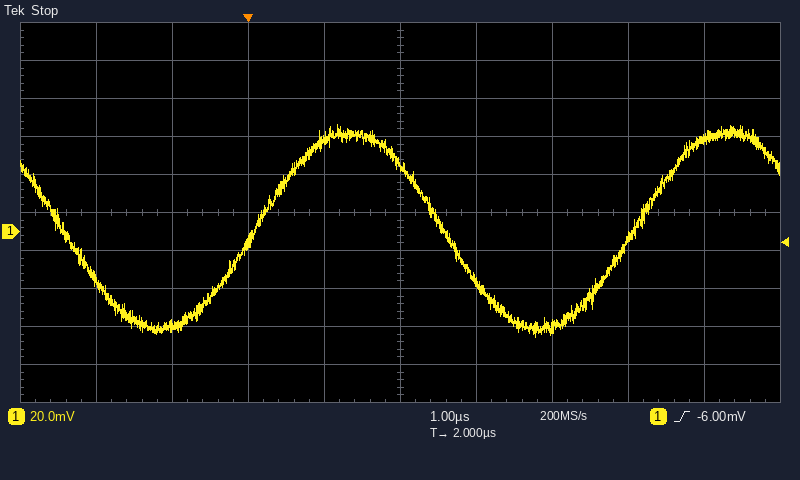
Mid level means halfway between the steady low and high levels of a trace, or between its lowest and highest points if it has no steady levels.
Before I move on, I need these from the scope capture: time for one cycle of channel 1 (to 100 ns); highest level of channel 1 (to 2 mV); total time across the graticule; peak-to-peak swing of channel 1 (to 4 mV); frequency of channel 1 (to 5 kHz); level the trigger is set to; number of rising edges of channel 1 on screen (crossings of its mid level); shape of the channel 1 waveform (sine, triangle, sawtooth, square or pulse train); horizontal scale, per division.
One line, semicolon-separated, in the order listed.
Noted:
5.0 µs; 56 mV; 10 µs; 112 mV; 200 kHz; -6.00 mV; 2; sine; 1 µs
